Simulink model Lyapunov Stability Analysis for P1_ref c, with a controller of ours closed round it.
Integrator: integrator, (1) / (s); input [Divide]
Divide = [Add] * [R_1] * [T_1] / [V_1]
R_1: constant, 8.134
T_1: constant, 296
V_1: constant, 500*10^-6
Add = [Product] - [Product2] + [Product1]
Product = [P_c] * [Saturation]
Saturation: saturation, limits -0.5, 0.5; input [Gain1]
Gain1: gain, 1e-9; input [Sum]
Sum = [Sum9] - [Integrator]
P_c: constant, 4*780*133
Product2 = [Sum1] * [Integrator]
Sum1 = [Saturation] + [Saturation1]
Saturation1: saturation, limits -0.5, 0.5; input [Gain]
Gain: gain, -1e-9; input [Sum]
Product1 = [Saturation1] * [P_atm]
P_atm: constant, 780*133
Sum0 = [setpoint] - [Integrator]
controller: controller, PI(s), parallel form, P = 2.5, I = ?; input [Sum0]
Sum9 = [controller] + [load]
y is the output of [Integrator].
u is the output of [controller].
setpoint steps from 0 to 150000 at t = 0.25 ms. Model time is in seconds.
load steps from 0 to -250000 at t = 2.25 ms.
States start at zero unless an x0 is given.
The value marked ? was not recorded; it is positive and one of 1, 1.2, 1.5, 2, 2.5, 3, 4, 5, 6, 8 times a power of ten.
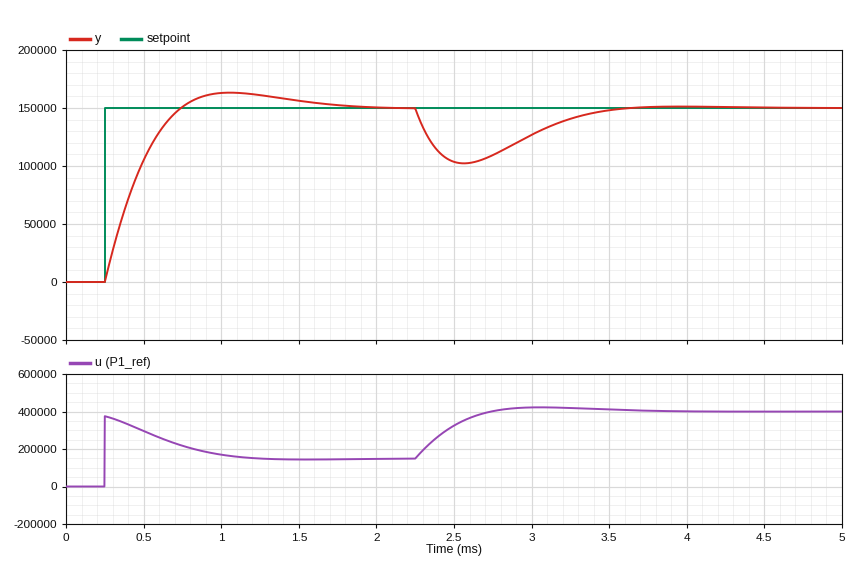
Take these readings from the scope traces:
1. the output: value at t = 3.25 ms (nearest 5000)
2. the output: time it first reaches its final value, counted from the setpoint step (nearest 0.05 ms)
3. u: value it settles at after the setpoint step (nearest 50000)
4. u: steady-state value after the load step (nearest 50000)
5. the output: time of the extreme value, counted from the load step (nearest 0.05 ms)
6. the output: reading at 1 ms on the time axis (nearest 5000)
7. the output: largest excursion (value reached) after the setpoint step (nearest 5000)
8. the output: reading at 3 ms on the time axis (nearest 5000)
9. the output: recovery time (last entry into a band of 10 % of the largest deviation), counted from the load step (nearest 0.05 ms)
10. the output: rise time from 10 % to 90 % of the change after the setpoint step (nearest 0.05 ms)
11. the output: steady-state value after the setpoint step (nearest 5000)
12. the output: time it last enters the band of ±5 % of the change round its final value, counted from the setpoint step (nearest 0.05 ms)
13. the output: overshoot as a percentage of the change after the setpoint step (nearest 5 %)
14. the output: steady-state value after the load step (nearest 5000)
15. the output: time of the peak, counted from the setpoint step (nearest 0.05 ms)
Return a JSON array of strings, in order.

["140000", "0.50 ms", "150000", "400000", "0.30 ms", "165000", "165000", "125000", "1.15 ms", "0.35 ms", "150000", "1.20 ms", "10 %", "150000", "0.80 ms"]
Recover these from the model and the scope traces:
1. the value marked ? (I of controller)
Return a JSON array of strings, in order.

["8000"]
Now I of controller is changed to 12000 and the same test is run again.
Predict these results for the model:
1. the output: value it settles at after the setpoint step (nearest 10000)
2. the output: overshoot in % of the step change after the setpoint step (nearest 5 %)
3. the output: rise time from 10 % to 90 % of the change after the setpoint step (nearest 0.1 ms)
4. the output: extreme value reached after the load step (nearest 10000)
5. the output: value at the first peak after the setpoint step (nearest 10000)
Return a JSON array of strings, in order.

["150000", "15 %", "0.3 ms", "110000", "170000"]
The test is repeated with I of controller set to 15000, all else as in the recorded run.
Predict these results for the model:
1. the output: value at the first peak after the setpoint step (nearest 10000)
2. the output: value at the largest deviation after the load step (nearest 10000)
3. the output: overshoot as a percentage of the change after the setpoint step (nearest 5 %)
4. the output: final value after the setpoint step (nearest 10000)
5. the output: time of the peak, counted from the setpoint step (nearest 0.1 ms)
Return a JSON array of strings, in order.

["180000", "110000", "20 %", "150000", "0.6 ms"]
